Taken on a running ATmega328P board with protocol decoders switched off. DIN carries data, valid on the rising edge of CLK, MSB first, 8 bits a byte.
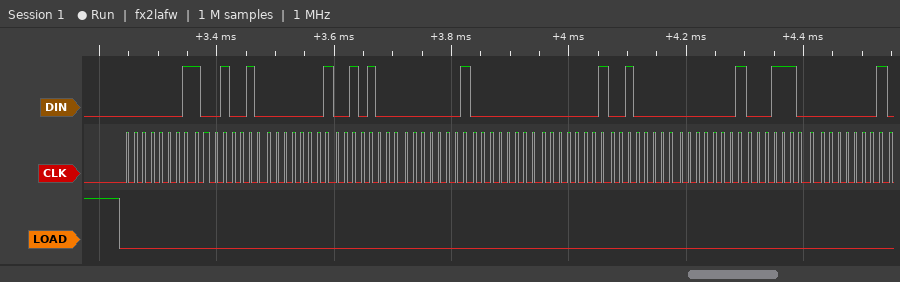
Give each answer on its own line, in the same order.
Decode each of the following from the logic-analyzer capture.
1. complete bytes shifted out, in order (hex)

01 92 01 28 01 00 01 20 01 1C 01
